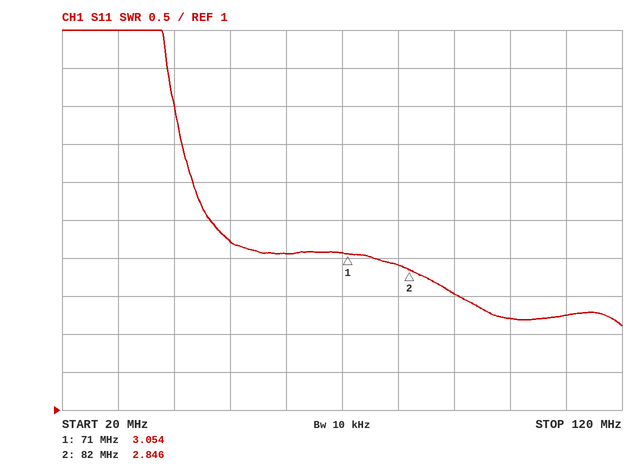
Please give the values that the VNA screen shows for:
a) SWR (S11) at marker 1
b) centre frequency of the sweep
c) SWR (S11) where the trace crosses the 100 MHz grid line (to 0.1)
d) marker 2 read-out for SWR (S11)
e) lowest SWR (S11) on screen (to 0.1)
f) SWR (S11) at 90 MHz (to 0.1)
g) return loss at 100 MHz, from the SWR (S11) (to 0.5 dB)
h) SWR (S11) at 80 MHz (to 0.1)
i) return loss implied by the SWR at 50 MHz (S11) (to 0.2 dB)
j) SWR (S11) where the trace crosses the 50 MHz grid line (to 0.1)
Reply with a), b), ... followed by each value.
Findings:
a) 3.054
b) 70 MHz
c) 2.2
d) 2.846
e) 2.1
f) 2.5
g) 8.5 dB
h) 2.9
i) 5.6 dB
j) 3.2
